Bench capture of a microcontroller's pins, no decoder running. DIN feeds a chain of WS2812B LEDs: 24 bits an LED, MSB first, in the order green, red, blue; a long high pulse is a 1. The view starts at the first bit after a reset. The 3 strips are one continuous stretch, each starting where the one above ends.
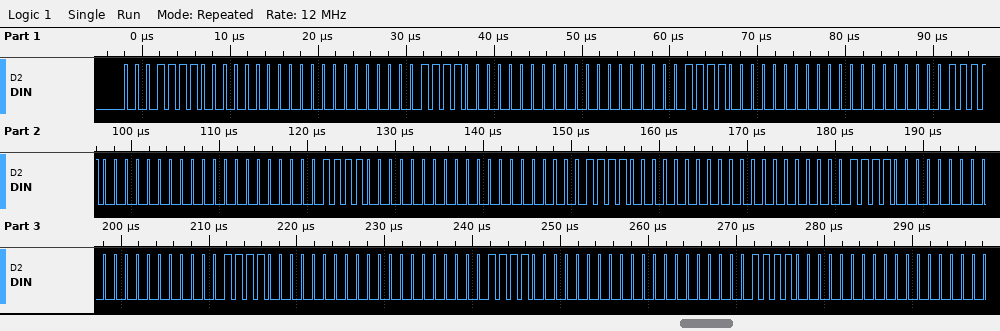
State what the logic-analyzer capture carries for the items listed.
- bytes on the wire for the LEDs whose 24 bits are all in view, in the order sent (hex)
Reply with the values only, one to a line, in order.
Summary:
1E 00 00 1E 00 00 1E 00 00 1E 00 00 1E 00 00 1E 00 00 1E 00 00 1E 00 00 1E 00 00 1E 00 00
